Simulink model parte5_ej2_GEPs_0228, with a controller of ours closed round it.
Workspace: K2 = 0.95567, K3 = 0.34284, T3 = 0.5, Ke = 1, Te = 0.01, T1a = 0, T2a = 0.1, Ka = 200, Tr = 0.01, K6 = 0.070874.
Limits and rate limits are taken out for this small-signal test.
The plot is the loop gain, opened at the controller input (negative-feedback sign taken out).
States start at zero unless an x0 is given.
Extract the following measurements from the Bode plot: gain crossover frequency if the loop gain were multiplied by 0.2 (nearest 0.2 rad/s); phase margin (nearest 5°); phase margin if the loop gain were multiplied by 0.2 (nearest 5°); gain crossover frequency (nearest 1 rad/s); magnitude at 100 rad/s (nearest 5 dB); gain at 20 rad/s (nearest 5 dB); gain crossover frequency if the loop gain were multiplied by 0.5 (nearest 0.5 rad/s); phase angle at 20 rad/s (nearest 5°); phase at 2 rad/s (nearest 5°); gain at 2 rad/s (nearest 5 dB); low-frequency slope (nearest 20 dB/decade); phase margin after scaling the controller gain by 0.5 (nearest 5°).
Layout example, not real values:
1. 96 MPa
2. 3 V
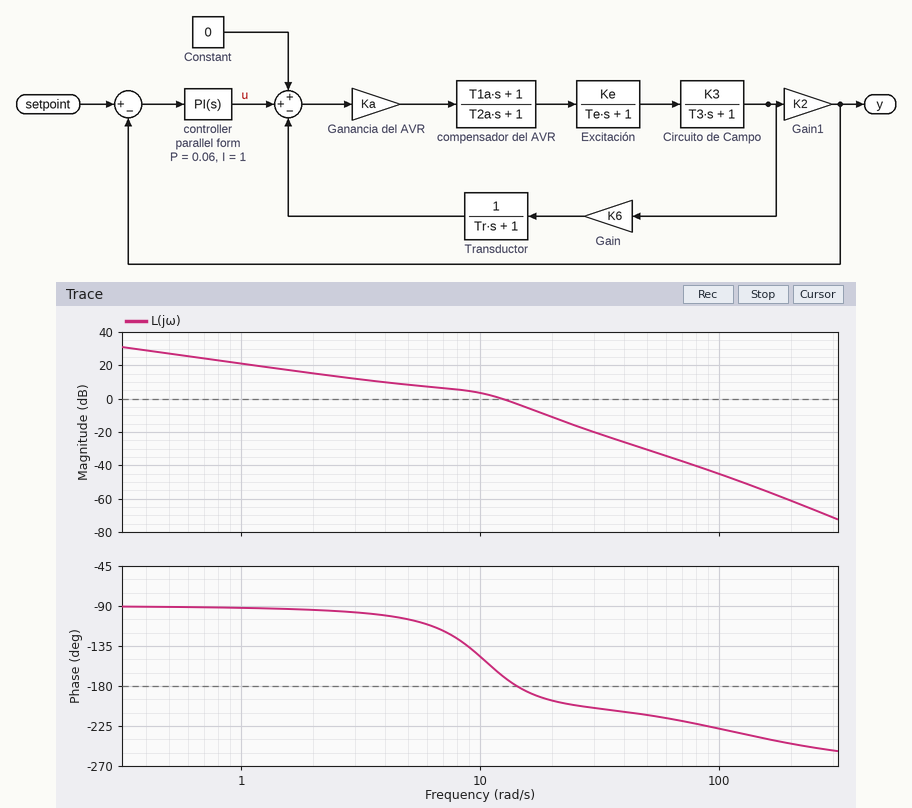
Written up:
1. 2.4 rad/s
2. 10°
3. 85°
4. 12 rad/s
5. -45 dB
6. -10 dB
7. 7.5 rad/s
8. -195°
9. -95°
10. 15 dB
11. -20 dB/decade
12. 60°
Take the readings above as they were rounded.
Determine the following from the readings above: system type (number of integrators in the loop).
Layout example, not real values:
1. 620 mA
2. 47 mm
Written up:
1. 1
